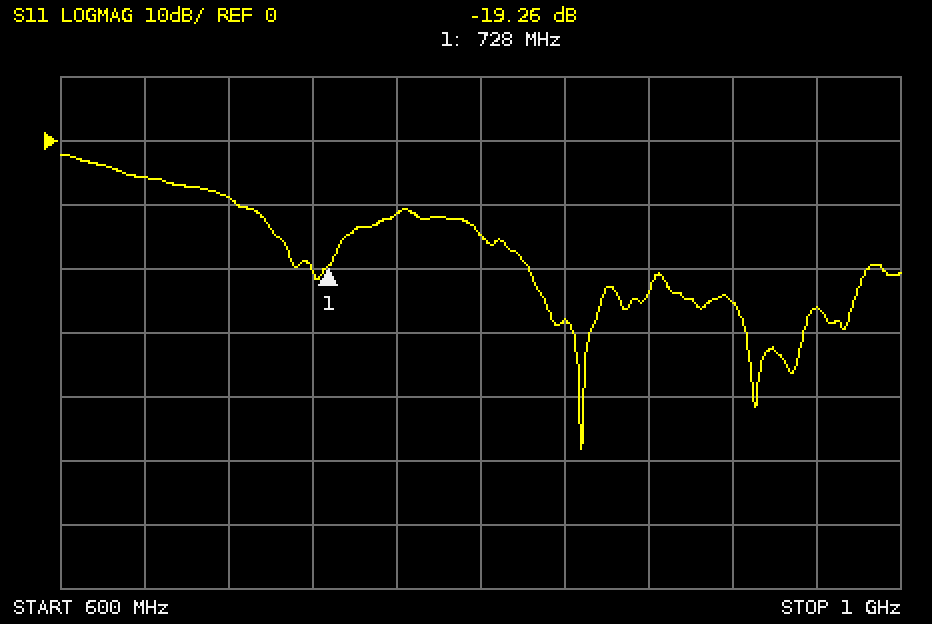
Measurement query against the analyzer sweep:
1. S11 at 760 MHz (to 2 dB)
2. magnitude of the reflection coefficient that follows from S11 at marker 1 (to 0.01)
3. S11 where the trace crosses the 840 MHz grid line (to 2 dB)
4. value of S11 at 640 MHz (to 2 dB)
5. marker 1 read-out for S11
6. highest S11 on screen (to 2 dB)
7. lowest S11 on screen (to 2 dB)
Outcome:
-12 dB
0.11
-28 dB
-6 dB
-19.26 dB
-2 dB
-48 dB
